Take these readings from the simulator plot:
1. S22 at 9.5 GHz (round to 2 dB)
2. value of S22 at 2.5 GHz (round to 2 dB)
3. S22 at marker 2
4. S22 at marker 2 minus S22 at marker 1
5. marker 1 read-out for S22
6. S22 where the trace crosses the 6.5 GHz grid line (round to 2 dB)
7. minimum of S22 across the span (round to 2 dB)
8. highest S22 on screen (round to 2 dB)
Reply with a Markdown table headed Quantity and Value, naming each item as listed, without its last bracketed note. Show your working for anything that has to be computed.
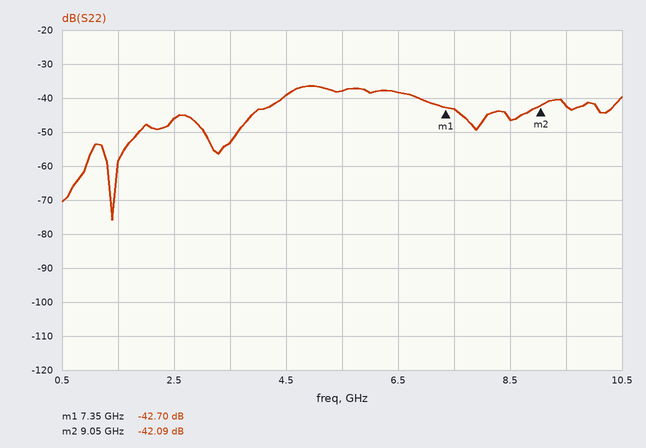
| Quantity | Value |
|---|---|
| S22 at 9.5 GHz | -42 dB |
| value of S22 at 2.5 GHz | -46 dB |
| S22 at marker 2 | -42.09 dB |
| S22 at marker 2 minus S22 at marker 1 | -42.09 − (-42.7) = 0.61 dB |
| marker 1 read-out for S22 | -42.70 dB |
| S22 where the trace crosses the 6.5 GHz grid line | -38 dB |
| minimum of S22 across the span | -76 dB |
| highest S22 on screen | -36 dB |
